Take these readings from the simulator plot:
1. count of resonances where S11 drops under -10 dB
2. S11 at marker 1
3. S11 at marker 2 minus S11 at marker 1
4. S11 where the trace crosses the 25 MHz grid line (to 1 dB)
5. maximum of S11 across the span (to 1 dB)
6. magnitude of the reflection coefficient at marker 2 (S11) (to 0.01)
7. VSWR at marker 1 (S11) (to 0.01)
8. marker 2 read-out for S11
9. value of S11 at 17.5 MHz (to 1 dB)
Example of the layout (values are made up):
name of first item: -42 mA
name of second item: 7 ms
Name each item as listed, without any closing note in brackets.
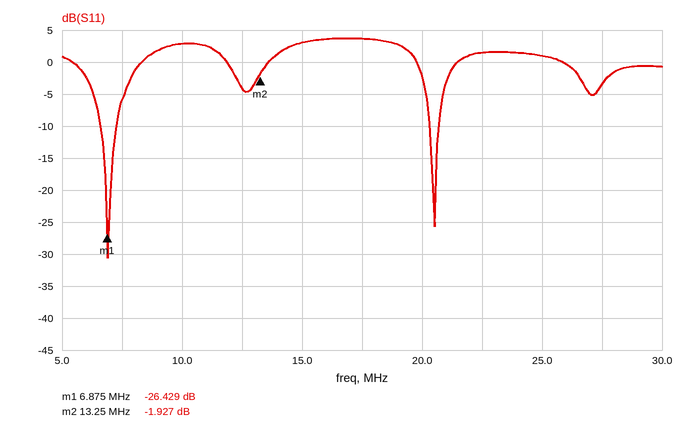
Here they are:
count of resonances where S11 drops under -10 dB: 2
S11 at marker 1: -26.429 dB
S11 at marker 2 minus S11 at marker 1: 24.502 dB
S11 where the trace crosses the 25 MHz grid line: 1 dB
maximum of S11 across the span: 4 dB
magnitude of the reflection coefficient at marker 2 (S11): 0.80
VSWR at marker 1 (S11): 1.10
marker 2 read-out for S11: -1.927 dB
value of S11 at 17.5 MHz: 4 dB
